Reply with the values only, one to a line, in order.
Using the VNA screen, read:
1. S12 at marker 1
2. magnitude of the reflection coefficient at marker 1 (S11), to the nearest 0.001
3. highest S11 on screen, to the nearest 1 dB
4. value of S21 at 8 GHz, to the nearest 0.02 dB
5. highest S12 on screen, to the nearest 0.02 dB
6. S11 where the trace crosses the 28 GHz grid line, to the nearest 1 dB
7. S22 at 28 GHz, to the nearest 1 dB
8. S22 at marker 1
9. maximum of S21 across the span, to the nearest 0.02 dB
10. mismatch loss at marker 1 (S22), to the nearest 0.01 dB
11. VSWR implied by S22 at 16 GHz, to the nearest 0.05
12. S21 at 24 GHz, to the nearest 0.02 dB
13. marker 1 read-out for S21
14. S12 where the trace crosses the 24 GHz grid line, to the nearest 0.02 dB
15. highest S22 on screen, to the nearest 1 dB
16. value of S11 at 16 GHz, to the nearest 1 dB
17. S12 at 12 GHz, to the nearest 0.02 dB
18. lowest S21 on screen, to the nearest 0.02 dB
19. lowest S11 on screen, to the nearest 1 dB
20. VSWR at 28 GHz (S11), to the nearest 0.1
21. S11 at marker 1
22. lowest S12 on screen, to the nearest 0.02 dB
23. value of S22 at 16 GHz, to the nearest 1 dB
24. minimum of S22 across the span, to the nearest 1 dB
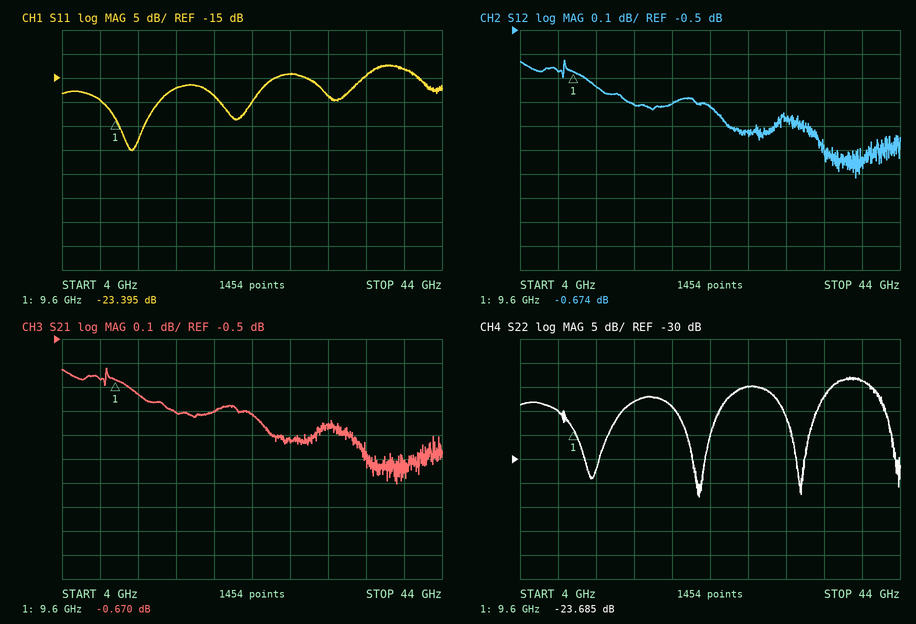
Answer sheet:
-0.674 dB
0.068
-12 dB
-0.66 dB
-0.62 dB
-14 dB
-15 dB
-23.685 dB
-0.62 dB
0.02 dB
1.30
-0.82 dB
-0.670 dB
-0.82 dB
-13 dB
-17 dB
-0.74 dB
-1.10 dB
-30 dB
1.5
-23.395 dB
-1.12 dB
-18 dB
-38 dB
